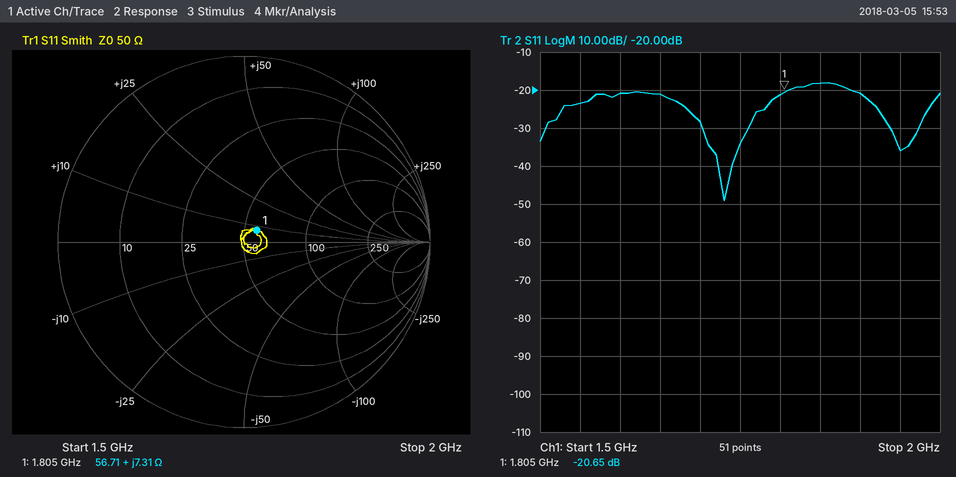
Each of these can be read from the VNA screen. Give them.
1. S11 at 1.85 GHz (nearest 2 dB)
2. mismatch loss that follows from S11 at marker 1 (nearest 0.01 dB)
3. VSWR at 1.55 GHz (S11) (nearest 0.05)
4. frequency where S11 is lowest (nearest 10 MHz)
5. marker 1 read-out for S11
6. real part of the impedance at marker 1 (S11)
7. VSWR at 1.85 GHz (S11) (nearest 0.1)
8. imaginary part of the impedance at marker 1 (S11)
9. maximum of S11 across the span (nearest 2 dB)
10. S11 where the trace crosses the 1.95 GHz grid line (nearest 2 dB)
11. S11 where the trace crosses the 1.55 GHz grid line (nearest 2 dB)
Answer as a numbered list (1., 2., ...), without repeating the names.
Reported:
1. -18 dB
2. 0.04 dB
3. 1.15
4. 1.73 GHz
5. -20.65 dB
6. 56.71 Ω
7. 1.3
8. +7.31 Ω
9. -18 dB
10. -36 dB
11. -24 dB
